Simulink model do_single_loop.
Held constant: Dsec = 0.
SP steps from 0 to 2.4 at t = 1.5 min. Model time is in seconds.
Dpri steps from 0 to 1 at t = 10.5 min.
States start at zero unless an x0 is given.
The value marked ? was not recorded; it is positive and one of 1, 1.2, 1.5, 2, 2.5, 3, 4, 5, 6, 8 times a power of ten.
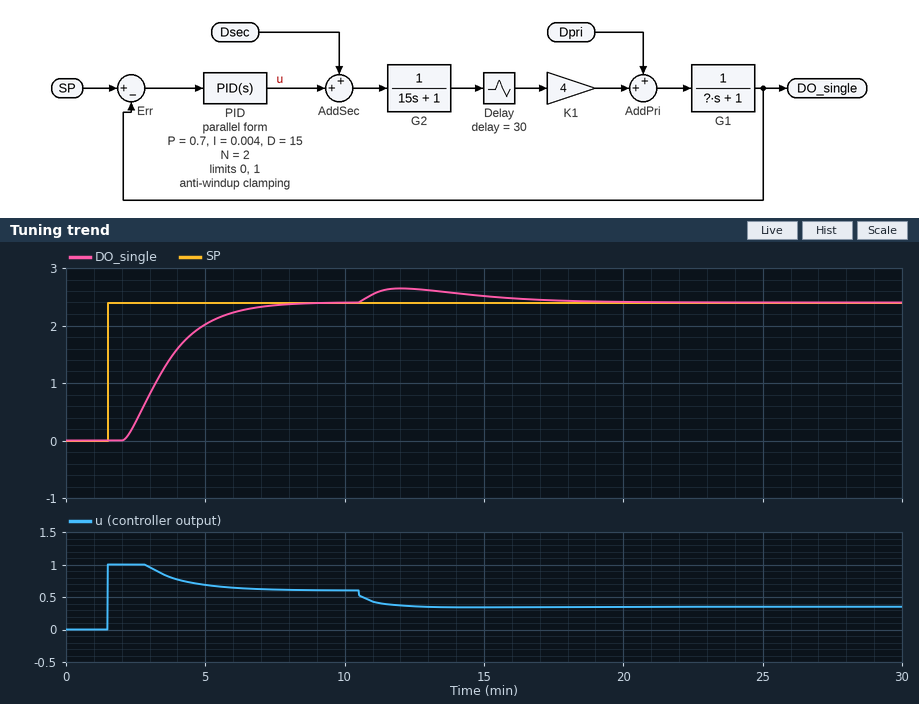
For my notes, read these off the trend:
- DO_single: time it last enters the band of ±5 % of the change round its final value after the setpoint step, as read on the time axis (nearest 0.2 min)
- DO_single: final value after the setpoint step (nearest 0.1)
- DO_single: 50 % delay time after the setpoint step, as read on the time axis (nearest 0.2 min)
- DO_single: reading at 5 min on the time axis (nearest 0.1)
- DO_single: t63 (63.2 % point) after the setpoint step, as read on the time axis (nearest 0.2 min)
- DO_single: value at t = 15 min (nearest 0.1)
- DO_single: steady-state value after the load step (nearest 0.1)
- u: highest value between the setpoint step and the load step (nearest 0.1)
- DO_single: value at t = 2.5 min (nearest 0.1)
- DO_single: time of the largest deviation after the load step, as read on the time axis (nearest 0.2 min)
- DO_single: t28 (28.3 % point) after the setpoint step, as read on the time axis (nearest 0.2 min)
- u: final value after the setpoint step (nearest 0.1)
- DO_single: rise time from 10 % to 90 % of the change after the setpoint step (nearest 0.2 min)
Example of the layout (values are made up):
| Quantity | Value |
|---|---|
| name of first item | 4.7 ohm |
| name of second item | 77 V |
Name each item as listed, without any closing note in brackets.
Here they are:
| Quantity | Value |
|---|---|
| DO_single: time it last enters the band of ±5 % of the change round its final value after the setpoint step, as read on the time axis | 6.4 min |
| DO_single: final value after the setpoint step | 2.4 |
| DO_single: 50 % delay time after the setpoint step, as read on the time axis | 3.4 min |
| DO_single: reading at 5 min on the time axis | 2.0 |
| DO_single: t63 (63.2 % point) after the setpoint step, as read on the time axis | 3.8 min |
| DO_single: value at t = 15 min | 2.5 |
| DO_single: steady-state value after the load step | 2.4 |
| u: highest value between the setpoint step and the load step | 1.0 |
| DO_single: value at t = 2.5 min | 0.3 |
| DO_single: time of the largest deviation after the load step, as read on the time axis | 12.0 min |
| DO_single: t28 (28.3 % point) after the setpoint step, as read on the time axis | 2.8 min |
| u: final value after the setpoint step | 0.6 |
| DO_single: rise time from 10 % to 90 % of the change after the setpoint step | 3.2 min |
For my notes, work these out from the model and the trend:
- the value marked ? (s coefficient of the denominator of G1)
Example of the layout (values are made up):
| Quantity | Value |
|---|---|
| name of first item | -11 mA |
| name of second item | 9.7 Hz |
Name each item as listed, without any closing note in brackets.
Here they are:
| Quantity | Value |
|---|---|
| the value marked ? | 200 |
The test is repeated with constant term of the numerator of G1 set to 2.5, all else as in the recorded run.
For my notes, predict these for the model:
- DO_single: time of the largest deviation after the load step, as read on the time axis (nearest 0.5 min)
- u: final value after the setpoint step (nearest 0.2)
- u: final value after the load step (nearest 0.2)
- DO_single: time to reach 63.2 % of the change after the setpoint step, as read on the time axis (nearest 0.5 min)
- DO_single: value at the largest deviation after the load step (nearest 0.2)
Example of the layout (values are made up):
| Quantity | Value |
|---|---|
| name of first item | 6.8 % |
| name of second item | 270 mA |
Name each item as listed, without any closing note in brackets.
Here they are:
| Quantity | Value |
|---|---|
| DO_single: time of the largest deviation after the load step, as read on the time axis | 11.5 min |
| u: final value after the setpoint step | 0.2 |
| u: final value after the load step | 0.0 |
| DO_single: time to reach 63.2 % of the change after the setpoint step, as read on the time axis | 3.0 min |
| DO_single: value at the largest deviation after the load step | 2.8 |
